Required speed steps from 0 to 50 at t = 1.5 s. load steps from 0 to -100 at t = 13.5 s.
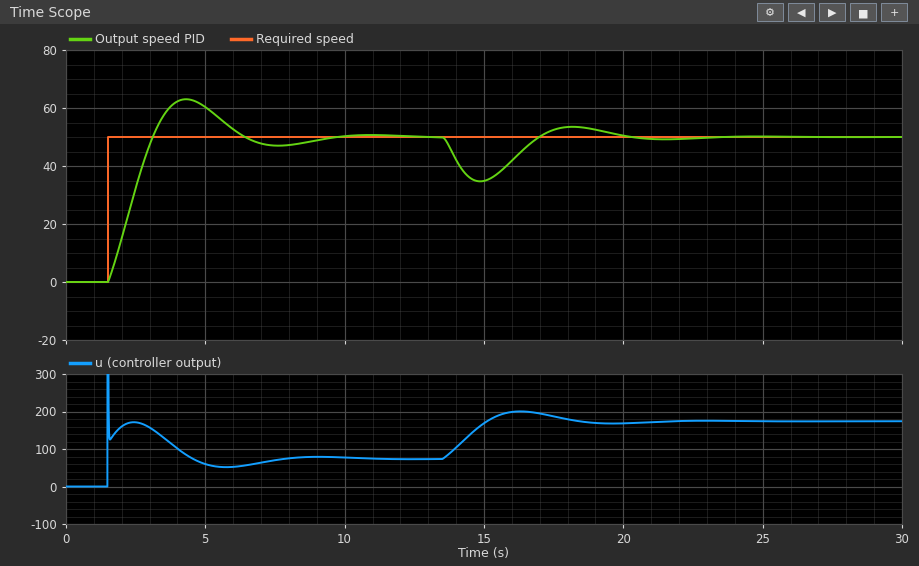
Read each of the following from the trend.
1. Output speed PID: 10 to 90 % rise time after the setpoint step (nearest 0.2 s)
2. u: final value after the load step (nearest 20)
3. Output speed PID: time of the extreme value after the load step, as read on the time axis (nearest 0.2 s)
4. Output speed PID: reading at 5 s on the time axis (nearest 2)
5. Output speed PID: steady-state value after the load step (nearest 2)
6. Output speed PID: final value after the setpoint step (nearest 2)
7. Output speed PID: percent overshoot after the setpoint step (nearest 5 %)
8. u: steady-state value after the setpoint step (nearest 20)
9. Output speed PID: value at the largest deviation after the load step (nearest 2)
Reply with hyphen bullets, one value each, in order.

- 1.2 s
- 180
- 14.8 s
- 60
- 50
- 50
- 25 %
- 80
- 34
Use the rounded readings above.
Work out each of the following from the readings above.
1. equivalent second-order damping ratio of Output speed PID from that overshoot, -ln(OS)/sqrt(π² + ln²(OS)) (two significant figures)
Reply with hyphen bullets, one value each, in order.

- 0.40
